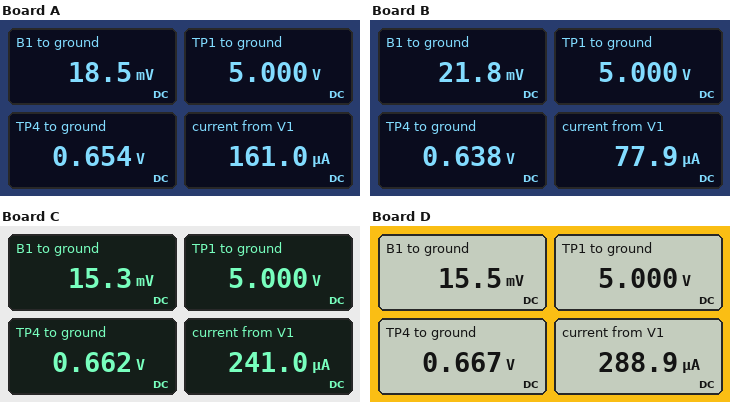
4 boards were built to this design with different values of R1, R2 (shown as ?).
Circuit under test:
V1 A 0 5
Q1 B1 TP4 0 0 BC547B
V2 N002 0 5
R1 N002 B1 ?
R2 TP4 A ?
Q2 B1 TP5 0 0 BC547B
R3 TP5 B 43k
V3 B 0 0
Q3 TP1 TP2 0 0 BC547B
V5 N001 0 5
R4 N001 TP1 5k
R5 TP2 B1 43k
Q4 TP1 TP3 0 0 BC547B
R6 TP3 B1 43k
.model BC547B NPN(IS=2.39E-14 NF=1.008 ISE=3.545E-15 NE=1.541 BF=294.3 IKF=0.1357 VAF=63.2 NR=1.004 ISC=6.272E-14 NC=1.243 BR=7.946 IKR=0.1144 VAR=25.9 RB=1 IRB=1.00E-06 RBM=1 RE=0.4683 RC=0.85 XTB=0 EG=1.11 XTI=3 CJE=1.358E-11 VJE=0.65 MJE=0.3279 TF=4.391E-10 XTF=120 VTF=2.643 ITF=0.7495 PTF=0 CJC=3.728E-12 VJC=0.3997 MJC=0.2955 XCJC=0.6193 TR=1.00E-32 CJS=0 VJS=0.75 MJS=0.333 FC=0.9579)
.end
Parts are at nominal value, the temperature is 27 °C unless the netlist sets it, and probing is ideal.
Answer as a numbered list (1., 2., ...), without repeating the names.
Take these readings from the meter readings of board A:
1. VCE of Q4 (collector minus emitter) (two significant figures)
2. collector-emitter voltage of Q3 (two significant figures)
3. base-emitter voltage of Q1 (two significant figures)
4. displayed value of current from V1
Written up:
1. 5.0 V
2. 5.0 V
3. 650 mV
4. 161.0 µA
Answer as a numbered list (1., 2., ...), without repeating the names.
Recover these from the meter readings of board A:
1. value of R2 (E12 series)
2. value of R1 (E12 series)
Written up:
1. 27 kΩ
2. 8.2 kΩ
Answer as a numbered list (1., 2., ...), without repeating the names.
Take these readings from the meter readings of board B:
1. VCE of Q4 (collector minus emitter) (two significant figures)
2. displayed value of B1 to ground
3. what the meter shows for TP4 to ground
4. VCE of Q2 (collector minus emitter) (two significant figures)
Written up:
1. 5.0 V
2. 21.8 mV
3. 0.638 V
4. 22 mV
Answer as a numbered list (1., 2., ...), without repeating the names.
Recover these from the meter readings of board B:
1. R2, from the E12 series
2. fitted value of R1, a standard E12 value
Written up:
1. 56 kΩ
2. 12 kΩ
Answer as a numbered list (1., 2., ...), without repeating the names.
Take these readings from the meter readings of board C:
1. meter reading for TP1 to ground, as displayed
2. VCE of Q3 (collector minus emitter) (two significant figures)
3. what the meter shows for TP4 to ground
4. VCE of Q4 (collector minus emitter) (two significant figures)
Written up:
1. 5.000 V
2. 5.0 V
3. 0.662 V
4. 5.0 V
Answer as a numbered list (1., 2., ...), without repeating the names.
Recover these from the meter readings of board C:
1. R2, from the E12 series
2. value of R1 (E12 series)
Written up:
1. 18 kΩ
2. 8.2 kΩ
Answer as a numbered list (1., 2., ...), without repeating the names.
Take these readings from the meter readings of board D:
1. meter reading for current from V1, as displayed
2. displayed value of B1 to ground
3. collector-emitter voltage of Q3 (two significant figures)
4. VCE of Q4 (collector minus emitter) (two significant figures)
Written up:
1. 288.9 µA
2. 15.5 mV
3. 5.0 V
4. 5.0 V
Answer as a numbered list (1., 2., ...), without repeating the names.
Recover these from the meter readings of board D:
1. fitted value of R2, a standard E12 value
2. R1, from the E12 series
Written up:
1. 15 kΩ
2. 6.8 kΩ
